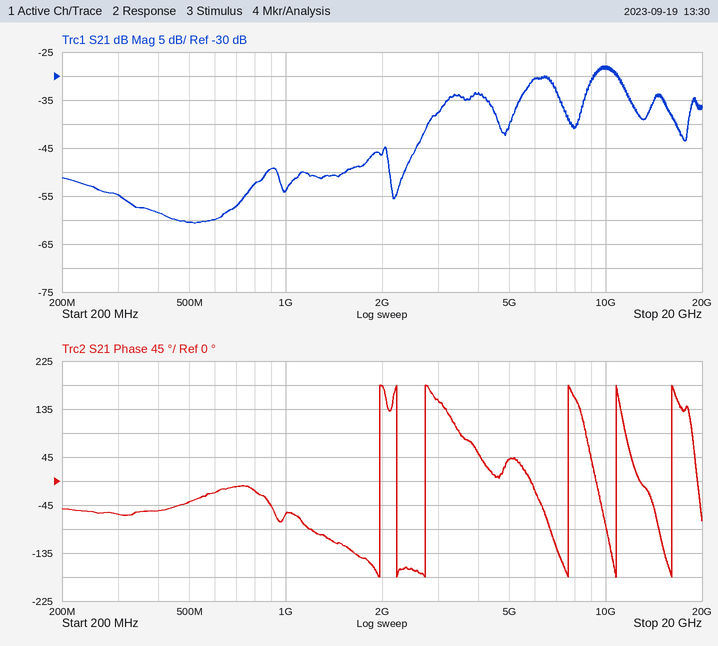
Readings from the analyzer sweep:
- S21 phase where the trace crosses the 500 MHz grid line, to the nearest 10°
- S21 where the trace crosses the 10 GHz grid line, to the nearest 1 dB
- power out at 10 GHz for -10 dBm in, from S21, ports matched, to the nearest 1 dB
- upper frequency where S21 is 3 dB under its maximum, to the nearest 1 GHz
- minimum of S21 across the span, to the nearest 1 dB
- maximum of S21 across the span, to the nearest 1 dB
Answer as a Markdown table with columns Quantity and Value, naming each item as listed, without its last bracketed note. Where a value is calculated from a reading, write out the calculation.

| Quantity | Value |
|---|---|
| S21 phase where the trace crosses the 500 MHz grid line, to the nearest 10° | -40° |
| S21 where the trace crosses the 10 GHz grid line, to the nearest 1 dB | -28 dB |
| power out at 10 GHz for -10 dBm in, from S21, ports matched, to the nearest 1 dB | -10 dBm + (-28 dB) = -38 dBm |
| upper frequency where S21 is 3 dB under its maximum, to the nearest 1 GHz | 11 GHz |
| minimum of S21 across the span, to the nearest 1 dB | -61 dB |
| maximum of S21 across the span, to the nearest 1 dB | -28 dB |
